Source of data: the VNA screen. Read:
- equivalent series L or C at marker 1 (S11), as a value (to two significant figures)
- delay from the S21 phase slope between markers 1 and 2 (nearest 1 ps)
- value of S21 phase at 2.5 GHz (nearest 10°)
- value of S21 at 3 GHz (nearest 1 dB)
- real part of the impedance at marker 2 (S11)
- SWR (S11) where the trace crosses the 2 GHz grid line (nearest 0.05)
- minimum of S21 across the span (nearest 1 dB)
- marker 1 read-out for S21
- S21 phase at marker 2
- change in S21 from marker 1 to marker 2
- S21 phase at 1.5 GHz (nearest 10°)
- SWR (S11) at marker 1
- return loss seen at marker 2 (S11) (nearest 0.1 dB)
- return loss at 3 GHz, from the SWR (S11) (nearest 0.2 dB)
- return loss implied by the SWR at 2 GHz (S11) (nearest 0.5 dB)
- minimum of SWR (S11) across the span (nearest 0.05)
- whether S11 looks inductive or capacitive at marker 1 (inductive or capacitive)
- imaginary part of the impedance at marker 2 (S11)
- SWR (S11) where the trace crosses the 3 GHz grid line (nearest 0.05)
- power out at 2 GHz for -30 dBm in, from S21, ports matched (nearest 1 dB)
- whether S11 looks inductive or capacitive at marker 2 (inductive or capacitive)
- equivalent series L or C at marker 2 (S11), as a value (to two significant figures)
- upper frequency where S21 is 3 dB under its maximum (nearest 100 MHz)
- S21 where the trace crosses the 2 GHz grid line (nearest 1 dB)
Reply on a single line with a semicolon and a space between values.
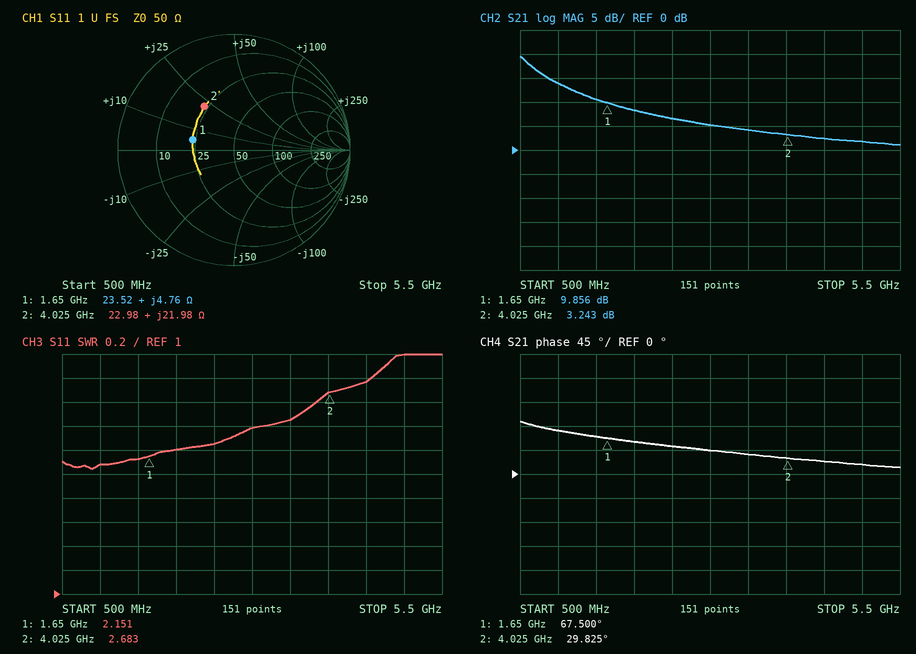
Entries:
460 pH; 44 ps; 50°; 5 dB; 22.98 Ω; 2.20; 1 dB; 9.856 dB; 29.825°; -6.613 dB; 70°; 2.151; 6.8 dB; 7.8 dB; 8.5 dB; 2.05; inductive; +21.98 Ω; 2.40; -22 dBm; inductive; 870 pH; 700 MHz; 8 dB
